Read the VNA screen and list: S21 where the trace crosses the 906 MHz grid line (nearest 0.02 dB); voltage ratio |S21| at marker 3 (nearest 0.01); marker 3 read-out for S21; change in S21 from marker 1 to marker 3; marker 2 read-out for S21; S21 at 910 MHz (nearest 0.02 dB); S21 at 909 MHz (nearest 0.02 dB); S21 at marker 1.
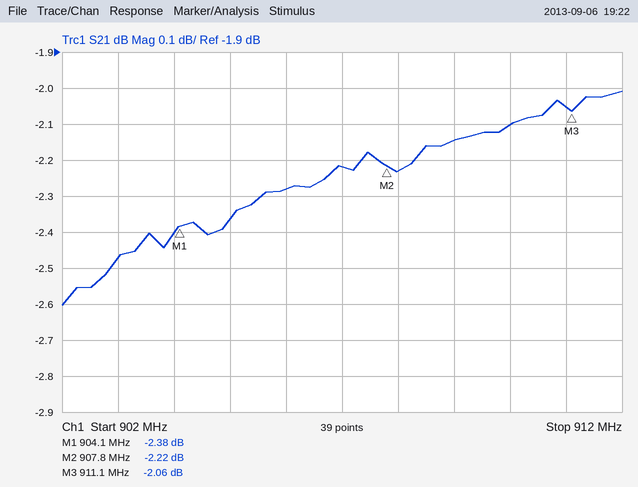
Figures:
-2.28 dB
0.79
-2.06 dB
0.32 dB
-2.22 dB
-2.10 dB
-2.14 dB
-2.38 dB
